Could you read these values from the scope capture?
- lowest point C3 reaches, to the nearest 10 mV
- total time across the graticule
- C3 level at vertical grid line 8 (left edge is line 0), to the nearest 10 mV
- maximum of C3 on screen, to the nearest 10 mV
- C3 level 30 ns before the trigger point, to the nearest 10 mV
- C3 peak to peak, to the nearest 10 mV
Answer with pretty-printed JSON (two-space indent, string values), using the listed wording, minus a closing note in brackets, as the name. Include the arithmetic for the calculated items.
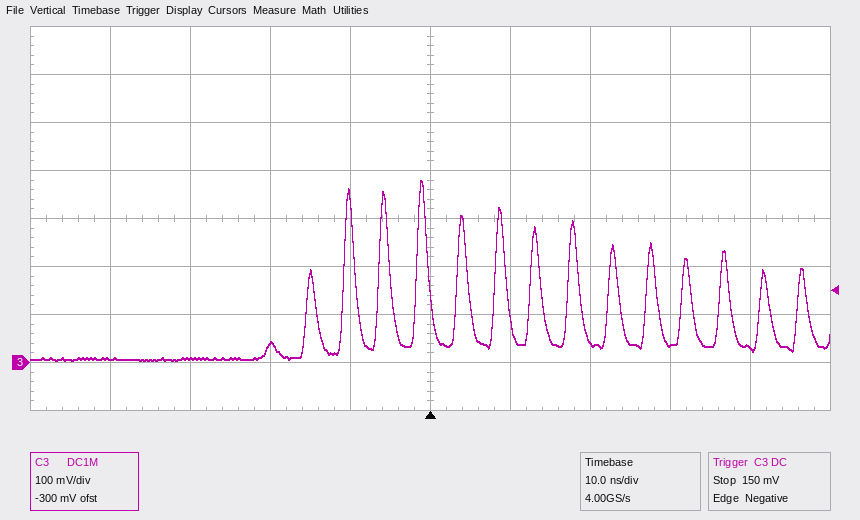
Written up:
{
  "lowest point C3 reaches, to the nearest 10 mV": "0 mV",
  "total time across the graticule": "100 ns",
  "C3 level at vertical grid line 8 (left edge is line 0), to the nearest 10 mV": "40 mV",
  "maximum of C3 on screen, to the nearest 10 mV": "380 mV",
  "C3 level 30 ns before the trigger point, to the nearest 10 mV": "10 mV",
  "C3 peak to peak, to the nearest 10 mV": "380 mV − (0 mV) = 380 mV"
}
